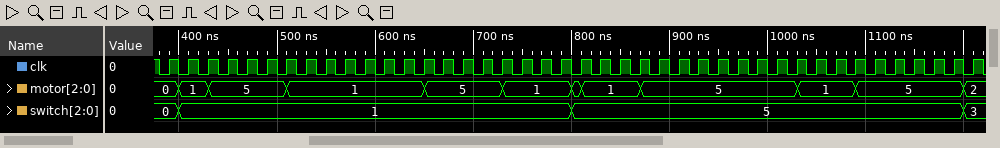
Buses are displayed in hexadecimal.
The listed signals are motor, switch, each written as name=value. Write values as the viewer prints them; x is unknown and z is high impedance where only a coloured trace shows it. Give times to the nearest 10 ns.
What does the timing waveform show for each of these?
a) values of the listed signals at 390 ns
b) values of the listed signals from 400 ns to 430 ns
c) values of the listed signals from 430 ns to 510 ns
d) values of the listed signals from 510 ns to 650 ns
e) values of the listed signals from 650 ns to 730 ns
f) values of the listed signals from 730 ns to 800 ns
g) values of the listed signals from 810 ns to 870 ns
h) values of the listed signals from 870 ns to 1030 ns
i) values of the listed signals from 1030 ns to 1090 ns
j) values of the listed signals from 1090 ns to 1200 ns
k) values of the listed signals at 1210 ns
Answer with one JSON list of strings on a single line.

["motor=0, switch=0", "motor=1, switch=1", "motor=5, switch=1", "motor=1, switch=1", "motor=5, switch=1", "motor=1, switch=1", "motor=1, switch=5", "motor=5, switch=5", "motor=1, switch=5", "motor=5, switch=5", "motor=2, switch=3"]
